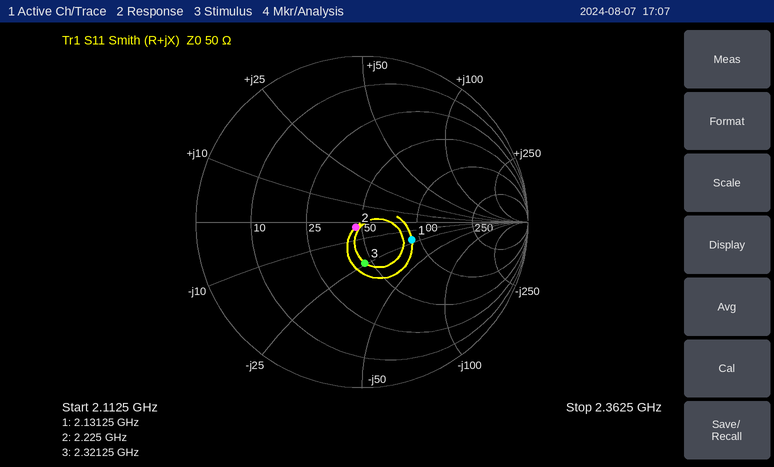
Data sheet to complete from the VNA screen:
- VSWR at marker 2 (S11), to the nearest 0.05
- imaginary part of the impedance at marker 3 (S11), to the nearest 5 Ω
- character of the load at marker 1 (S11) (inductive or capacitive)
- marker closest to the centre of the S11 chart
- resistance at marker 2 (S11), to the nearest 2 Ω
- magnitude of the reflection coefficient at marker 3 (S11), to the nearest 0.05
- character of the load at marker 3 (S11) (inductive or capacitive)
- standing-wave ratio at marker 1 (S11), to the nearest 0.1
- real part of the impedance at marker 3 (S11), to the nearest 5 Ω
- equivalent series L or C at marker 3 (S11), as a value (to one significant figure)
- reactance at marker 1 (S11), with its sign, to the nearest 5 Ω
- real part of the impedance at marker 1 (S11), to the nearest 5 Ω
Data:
1.10
-25 Ω
capacitive
marker 2
46 Ω
0.25
capacitive
1.9
45 Ω
3 pF
-20 Ω
90 Ω
